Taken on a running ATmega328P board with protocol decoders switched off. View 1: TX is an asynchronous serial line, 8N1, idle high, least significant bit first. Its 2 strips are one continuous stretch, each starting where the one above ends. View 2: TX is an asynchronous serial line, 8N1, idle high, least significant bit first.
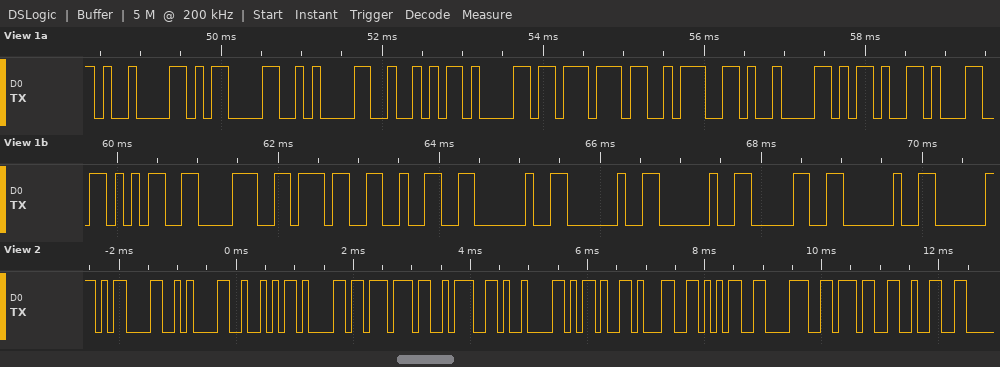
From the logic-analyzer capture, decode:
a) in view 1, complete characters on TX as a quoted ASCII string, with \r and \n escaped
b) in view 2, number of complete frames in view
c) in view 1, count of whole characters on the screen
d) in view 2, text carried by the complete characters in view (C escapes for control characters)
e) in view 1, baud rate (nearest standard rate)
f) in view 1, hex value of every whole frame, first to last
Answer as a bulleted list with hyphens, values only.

- "\t\r\nRaw:\t-15872   0 "
- 13
- 19
- "\r\nRaw:\t-15872"
- 9600 baud
- 09 0D 0A 52 61 77 3A 09 2D 31 35 38 37 32 20 20 20 30 20
